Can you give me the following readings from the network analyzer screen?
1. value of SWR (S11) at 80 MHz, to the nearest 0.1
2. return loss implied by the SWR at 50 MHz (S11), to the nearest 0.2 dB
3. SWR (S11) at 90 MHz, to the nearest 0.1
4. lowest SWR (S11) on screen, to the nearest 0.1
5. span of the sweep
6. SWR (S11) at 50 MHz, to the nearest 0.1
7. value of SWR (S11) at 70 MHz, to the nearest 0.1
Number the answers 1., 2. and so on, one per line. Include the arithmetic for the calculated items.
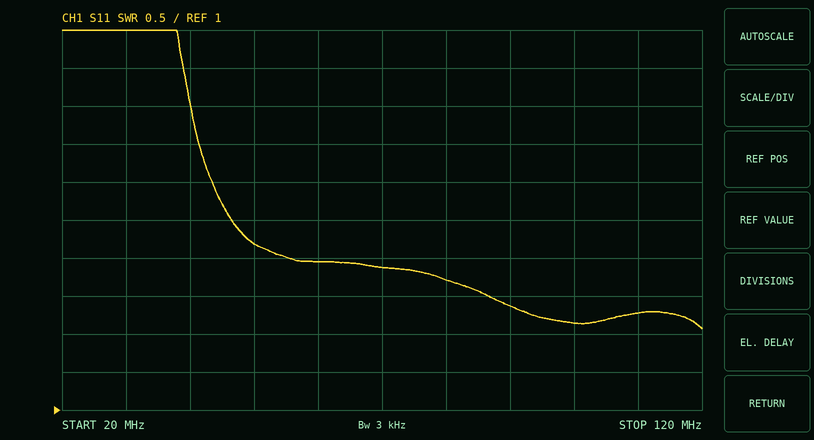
1. 2.7
2. −20 log10((3.2 − 1)/(3.2 + 1)) ≈ 5.6 dB
3. 2.4
4. 2.1
5. 100 MHz
6. 3.2
7. 2.9
